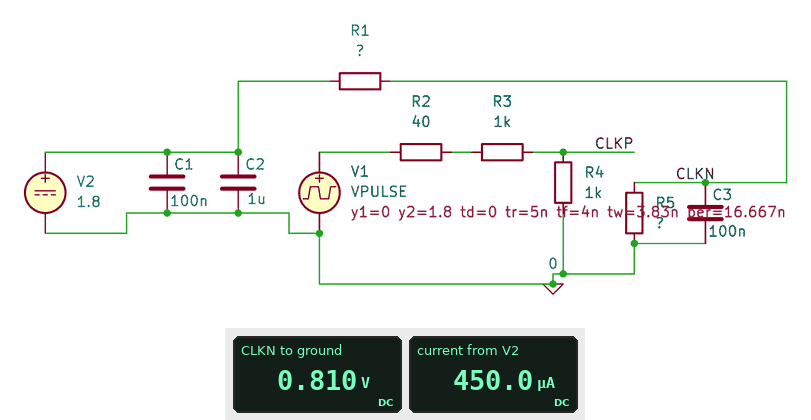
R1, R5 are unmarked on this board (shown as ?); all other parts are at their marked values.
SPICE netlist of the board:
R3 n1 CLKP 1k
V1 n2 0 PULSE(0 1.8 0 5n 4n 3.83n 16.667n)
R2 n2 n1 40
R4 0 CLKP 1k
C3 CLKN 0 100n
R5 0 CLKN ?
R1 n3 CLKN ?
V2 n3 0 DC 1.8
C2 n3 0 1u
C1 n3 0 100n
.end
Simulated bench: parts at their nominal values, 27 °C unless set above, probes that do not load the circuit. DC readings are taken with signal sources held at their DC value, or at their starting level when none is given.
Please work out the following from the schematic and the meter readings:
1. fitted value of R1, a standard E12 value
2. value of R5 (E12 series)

2.2 kΩ
1.8 kΩ
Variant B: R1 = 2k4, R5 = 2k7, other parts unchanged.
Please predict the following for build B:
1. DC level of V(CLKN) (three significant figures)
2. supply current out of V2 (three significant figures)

953 mV
353 µA
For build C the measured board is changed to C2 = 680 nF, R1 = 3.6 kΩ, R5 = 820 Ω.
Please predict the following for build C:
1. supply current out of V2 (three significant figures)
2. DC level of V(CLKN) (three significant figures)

407 µA
334 mV
